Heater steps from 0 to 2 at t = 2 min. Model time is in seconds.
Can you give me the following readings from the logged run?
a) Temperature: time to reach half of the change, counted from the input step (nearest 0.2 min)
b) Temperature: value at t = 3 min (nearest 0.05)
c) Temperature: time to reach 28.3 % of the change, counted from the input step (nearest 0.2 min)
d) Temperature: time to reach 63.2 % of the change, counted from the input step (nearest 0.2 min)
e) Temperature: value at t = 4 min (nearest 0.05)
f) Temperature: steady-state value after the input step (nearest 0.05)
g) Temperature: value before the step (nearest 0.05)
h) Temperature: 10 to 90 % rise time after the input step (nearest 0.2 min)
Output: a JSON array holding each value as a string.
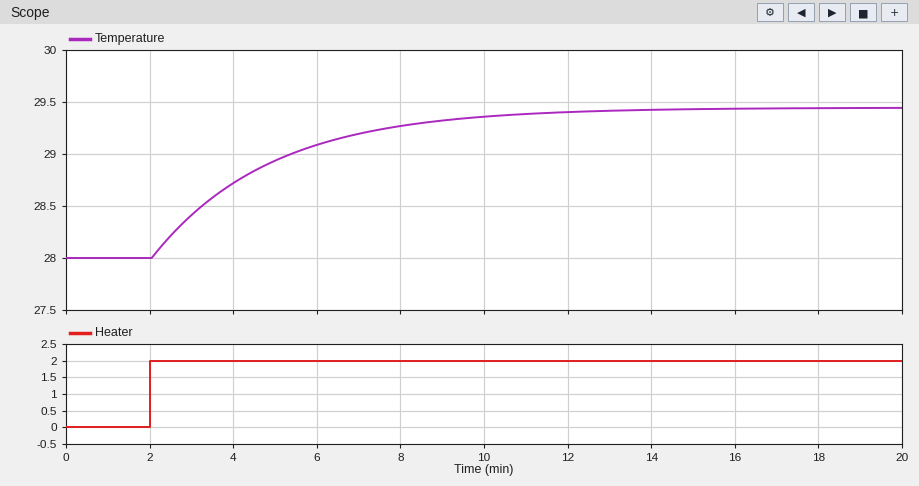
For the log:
["2.0 min", "28.40", "1.0 min", "2.8 min", "28.70", "29.45", "28.00", "6.2 min"]
